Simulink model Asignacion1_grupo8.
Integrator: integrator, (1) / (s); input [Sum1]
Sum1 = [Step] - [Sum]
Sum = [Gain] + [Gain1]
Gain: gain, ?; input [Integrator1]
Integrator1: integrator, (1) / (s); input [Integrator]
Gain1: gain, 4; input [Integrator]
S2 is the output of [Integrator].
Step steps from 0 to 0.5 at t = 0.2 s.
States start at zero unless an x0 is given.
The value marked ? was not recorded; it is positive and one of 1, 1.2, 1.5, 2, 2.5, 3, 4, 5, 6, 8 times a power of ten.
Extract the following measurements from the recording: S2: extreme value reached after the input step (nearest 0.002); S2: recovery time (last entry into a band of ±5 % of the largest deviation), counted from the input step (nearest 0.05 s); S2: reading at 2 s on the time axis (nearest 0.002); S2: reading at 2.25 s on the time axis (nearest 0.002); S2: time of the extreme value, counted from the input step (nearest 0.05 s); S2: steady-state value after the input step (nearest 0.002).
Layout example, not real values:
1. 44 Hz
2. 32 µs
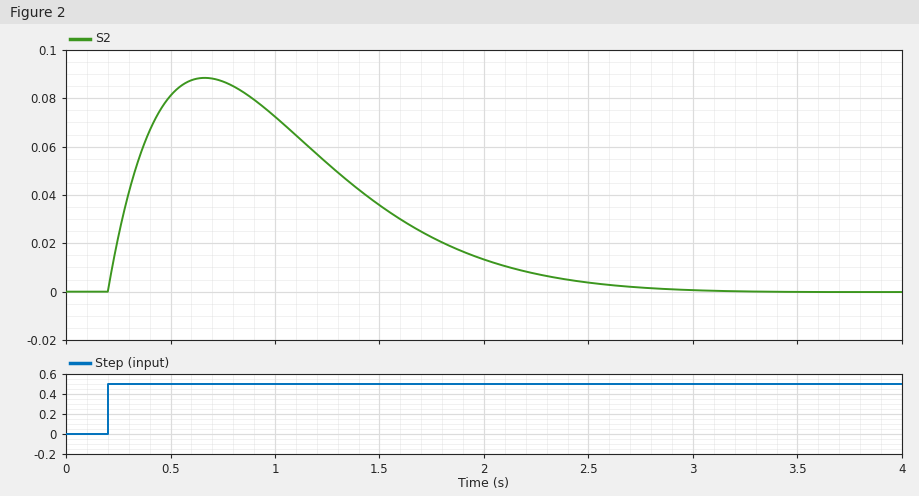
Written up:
1. 0.088
2. 2.25 s
3. 0.014
4. 0.008
5. 0.45 s
6. 0.000
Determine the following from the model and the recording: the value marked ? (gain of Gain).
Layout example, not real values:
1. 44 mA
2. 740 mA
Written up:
1. 5
